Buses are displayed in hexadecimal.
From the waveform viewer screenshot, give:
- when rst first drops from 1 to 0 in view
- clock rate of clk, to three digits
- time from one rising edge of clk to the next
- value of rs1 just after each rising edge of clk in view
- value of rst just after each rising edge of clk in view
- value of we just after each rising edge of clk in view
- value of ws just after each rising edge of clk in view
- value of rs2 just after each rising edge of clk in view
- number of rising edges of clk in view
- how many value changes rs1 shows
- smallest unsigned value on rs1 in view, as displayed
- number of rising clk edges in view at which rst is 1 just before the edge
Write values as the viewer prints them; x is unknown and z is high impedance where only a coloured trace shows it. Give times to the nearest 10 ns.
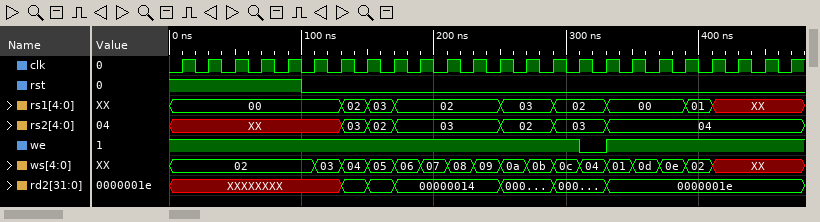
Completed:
100 ns
50.0 MHz
20 ns
00, 00, 00, 00, 00, 00, 02, 03, 02, 02, 02, 02, 03, 03, 02, 02, 00, 00, 00, 01, XX, XX, XX, XX
1 1 1 1 1 0 0 0 0 0 0 0 0 0 0 0 0 0 0 0 0 0 0 0
1 1 1 1 1 1 1 1 1 1 1 1 1 1 1 0 1 1 1 1 1 1 1 1
02, 02, 02, 02, 02, 03, 04, 05, 06, 07, 08, 09, 0a, 0b, 0c, 04, 01, 0d, 0e, 02, XX, XX, XX, XX
XX, XX, XX, XX, XX, XX, 03, 02, 03, 03, 03, 03, 02, 02, 03, 03, 04, 04, 04, 04, 04, 04, 04, 04
24
8
00
5
